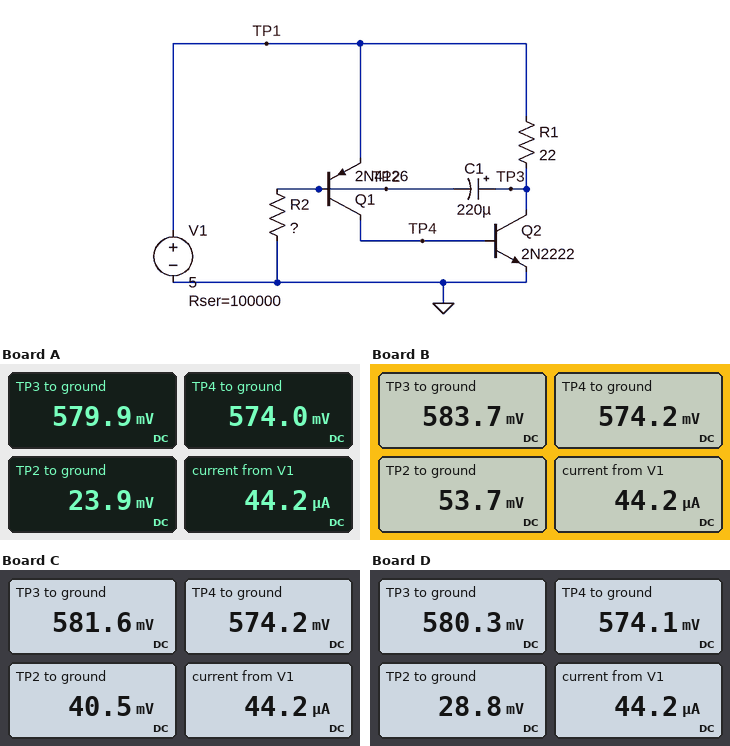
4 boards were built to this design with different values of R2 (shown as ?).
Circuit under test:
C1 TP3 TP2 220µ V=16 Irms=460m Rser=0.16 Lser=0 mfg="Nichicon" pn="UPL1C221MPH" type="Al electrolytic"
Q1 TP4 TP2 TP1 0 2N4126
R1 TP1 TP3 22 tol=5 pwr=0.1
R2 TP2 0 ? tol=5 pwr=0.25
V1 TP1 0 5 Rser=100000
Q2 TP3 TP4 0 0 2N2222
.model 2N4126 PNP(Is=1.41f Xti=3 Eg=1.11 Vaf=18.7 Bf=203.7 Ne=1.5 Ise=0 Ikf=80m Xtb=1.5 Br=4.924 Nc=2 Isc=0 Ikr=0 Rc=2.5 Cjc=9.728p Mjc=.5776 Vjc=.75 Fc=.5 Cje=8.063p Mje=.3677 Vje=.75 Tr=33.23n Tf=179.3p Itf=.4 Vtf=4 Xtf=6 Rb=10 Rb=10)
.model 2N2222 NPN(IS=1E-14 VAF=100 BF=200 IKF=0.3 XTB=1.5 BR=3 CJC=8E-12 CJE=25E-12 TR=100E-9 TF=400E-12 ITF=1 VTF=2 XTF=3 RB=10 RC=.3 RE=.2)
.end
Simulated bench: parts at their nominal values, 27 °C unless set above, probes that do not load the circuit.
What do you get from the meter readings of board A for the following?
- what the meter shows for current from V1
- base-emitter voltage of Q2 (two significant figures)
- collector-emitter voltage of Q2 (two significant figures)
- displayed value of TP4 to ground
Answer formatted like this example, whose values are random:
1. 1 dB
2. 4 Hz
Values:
1. 44.2 µA
2. 570 mV
3. 580 mV
4. 574.0 mV
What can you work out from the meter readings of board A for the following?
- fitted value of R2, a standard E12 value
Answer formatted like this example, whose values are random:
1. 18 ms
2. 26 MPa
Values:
1. 47 kΩ
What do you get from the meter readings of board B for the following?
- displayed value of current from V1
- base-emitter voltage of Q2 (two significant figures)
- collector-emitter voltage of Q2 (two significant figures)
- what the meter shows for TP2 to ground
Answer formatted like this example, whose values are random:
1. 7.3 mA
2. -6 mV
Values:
1. 44.2 µA
2. 570 mV
3. 580 mV
4. 53.7 mV
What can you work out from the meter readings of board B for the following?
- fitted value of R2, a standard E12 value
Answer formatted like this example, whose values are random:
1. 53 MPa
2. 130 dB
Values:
1. 330 kΩ
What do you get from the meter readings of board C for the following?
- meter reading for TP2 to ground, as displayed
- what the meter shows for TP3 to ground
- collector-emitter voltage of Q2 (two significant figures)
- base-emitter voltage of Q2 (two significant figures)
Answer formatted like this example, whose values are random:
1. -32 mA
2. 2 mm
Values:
1. 40.5 mV
2. 581.6 mV
3. 580 mV
4. 570 mV
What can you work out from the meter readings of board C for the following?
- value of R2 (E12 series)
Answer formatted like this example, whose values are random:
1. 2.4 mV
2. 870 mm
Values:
1. 150 kΩ
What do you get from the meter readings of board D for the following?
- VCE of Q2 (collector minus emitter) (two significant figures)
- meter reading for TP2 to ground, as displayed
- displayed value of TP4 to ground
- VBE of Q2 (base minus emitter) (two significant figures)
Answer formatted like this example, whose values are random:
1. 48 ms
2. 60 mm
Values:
1. 580 mV
2. 28.8 mV
3. 574.1 mV
4. 570 mV
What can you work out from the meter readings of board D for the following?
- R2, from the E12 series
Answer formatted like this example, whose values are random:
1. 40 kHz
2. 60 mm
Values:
1. 68 kΩ
